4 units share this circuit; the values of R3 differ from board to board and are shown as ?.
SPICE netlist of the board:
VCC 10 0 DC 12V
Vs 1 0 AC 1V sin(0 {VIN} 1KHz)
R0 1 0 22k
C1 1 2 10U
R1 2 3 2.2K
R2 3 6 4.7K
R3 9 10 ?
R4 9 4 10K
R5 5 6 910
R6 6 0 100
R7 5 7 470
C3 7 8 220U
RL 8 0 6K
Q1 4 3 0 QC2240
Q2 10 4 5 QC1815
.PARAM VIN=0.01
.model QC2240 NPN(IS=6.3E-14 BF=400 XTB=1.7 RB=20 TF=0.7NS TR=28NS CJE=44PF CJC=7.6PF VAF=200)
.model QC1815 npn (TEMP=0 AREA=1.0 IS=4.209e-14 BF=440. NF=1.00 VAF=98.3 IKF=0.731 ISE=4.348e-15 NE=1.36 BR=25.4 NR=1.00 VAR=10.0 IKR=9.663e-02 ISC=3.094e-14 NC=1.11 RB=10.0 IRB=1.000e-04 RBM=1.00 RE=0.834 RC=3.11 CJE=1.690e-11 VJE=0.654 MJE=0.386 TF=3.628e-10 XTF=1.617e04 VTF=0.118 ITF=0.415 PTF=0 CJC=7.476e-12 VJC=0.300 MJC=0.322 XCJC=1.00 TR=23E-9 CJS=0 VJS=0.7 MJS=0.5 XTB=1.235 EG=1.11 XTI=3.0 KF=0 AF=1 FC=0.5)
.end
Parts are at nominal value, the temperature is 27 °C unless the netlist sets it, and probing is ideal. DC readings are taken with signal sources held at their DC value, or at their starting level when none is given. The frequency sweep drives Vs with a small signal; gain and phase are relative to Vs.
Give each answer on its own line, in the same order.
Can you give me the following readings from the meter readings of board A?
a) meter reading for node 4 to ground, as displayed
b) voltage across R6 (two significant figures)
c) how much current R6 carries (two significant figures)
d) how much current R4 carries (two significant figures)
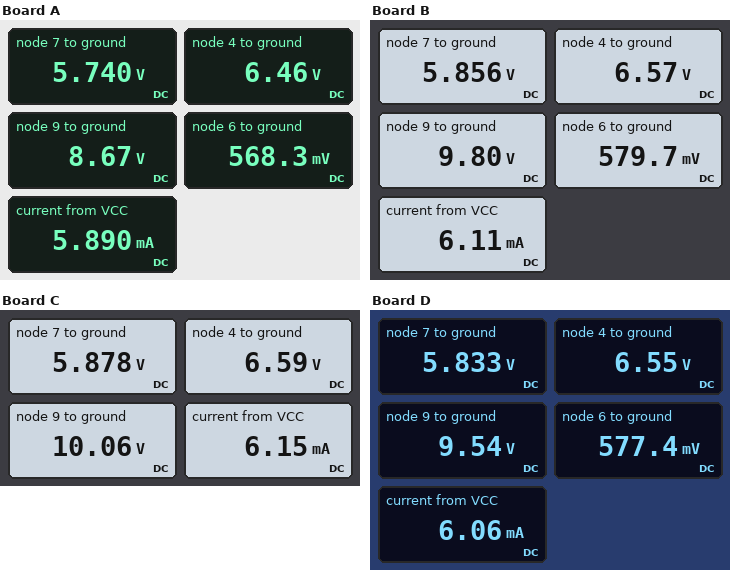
6.46 V
570 mV
5.7 mA
220 µA
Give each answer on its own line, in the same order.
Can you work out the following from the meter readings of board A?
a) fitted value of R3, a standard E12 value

15 kΩ
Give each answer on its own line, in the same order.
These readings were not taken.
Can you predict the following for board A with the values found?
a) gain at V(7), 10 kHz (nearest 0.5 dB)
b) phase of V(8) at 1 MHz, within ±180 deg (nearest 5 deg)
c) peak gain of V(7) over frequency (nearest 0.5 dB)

24.5 dB
125 deg
24.5 dB
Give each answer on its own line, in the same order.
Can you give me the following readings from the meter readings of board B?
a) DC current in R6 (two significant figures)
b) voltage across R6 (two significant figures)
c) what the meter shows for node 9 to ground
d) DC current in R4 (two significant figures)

5.8 mA
580 mV
9.80 V
320 µA
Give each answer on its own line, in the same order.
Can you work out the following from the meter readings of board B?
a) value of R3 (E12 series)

6.8 kΩ
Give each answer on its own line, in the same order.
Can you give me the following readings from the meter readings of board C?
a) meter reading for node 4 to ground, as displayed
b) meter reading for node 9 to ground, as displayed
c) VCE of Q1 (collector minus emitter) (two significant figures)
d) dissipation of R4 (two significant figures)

6.59 V
10.06 V
6.6 V
1.2 mW
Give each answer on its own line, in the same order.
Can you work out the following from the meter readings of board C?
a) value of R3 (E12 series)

5.6 kΩ
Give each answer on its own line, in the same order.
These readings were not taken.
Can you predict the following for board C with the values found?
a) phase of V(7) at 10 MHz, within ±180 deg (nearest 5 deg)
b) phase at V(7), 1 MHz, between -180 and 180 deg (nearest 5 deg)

60 deg
130 deg
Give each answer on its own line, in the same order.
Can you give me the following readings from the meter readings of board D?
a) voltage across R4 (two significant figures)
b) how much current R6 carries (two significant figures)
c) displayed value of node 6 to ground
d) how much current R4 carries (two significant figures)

3.0 V
5.8 mA
577.4 mV
300 µA
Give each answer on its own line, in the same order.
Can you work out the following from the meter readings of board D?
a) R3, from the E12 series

8.2 kΩ
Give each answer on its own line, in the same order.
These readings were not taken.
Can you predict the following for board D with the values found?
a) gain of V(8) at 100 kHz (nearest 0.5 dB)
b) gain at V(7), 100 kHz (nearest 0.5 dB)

24.5 dB
24.5 dB
